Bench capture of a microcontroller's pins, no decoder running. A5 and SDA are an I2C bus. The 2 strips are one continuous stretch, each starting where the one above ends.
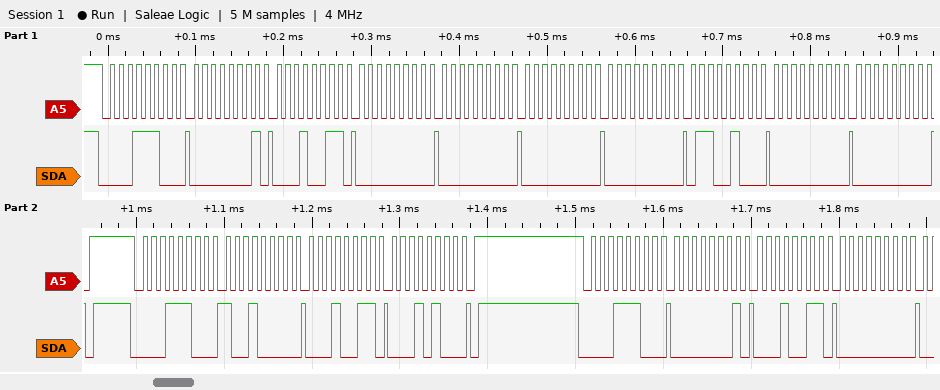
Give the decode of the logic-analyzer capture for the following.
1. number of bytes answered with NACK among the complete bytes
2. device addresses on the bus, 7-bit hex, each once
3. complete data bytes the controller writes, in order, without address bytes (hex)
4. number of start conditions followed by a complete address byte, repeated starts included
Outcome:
0
0x0E
01 13 00 00 00 00 64 00 00 90 13 14 01 13 00
3
